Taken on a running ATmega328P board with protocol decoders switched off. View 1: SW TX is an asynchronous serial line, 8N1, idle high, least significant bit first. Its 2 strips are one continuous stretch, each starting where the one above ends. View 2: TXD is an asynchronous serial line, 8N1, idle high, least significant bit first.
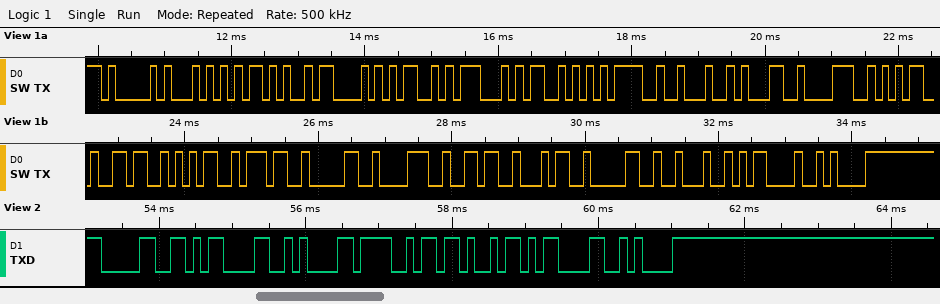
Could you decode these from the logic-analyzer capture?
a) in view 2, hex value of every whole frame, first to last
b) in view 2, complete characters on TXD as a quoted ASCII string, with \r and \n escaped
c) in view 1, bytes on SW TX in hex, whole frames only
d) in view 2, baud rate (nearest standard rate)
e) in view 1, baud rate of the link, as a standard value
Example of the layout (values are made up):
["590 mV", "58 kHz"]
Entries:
["30 0D 0A 4F 4B 0D 0A", "\"0\\r\\nOK\\r\\n\"", "41 54 2B 43 4D 47 53 3D 22 31 38 35 36 35 37 30 38 36 34 30 22 0D 0A", "9600 baud", "9600 baud"]
